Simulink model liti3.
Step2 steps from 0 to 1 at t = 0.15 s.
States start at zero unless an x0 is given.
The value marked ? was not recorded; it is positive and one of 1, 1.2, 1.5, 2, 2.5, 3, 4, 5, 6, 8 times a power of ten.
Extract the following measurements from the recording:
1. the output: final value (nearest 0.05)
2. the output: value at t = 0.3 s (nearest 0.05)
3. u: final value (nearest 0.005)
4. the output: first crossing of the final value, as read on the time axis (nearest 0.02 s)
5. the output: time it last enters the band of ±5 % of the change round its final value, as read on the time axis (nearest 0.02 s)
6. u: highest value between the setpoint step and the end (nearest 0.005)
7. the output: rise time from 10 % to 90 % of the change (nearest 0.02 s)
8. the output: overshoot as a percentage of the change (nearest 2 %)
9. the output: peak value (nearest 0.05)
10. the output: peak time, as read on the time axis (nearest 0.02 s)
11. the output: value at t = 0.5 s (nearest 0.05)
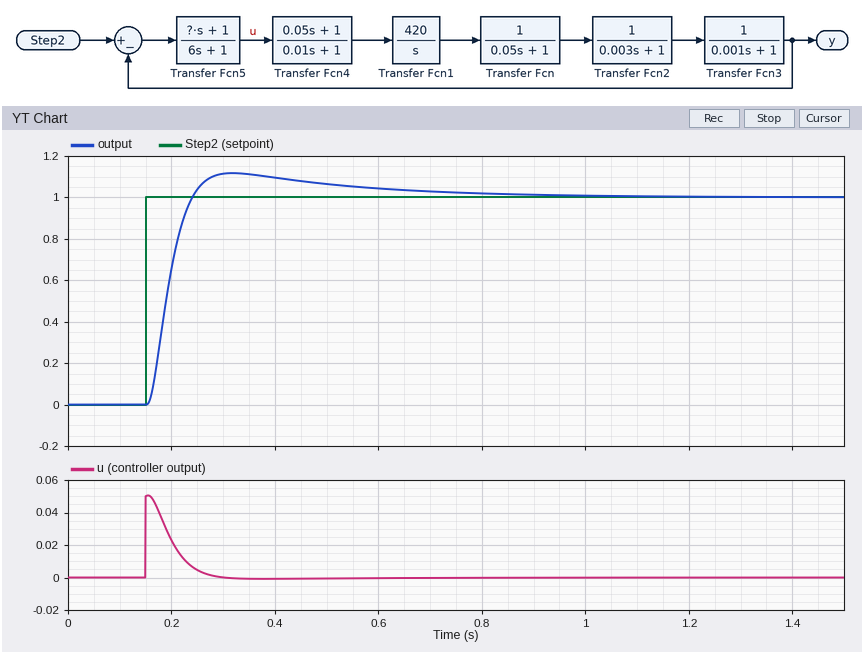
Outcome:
1.00
1.10
0.000
0.24 s
0.56 s
0.050
0.06 s
12 %
1.10
0.32 s
1.05
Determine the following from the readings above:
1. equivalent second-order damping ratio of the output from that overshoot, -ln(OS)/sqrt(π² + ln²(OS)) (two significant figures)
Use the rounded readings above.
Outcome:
0.56
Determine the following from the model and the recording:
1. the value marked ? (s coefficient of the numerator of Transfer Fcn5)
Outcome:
0.3
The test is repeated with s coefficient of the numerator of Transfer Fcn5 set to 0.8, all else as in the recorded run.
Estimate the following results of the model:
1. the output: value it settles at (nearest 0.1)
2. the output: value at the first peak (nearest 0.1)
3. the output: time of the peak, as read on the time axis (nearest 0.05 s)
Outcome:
1.0
1.2
0.20 s
